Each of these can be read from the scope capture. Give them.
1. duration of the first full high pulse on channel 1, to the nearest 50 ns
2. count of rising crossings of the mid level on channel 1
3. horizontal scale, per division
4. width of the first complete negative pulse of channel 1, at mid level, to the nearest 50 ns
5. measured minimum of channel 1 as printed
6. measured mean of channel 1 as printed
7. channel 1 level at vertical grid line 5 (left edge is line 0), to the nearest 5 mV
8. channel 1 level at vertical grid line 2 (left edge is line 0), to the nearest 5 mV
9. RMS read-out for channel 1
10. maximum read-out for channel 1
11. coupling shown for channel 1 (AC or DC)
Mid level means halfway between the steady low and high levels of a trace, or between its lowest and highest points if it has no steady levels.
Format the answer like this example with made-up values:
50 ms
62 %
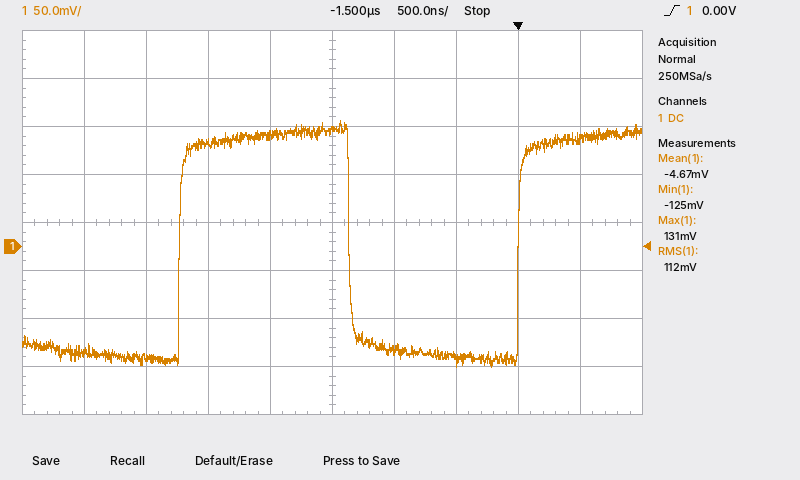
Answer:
1.35 µs
2
500 ns
1.35 µs
-125 mV
-4.67 mV
120 mV
-115 mV
112 mV
131 mV
DC
